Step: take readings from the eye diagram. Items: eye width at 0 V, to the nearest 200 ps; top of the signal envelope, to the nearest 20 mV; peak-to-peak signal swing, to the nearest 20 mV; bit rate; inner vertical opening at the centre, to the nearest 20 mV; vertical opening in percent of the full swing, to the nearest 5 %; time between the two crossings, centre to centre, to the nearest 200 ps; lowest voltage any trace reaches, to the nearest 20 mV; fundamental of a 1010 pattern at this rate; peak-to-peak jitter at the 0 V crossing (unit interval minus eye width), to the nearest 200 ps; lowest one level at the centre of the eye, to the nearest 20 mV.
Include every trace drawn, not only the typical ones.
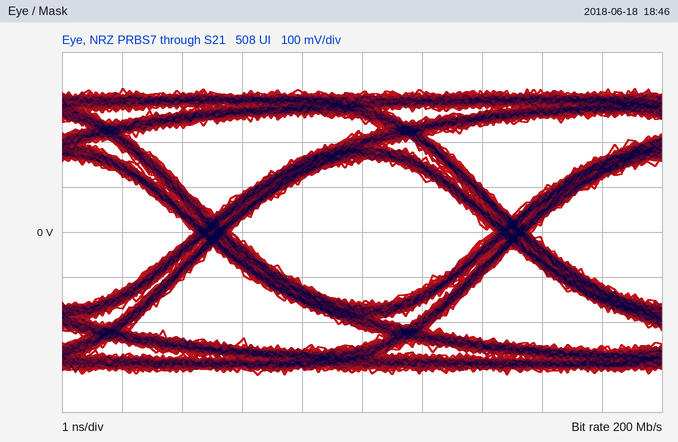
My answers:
4.4 ns
320 mV
640 mV
200 Mb/s
320 mV
50 %
5.0 ns
-320 mV
100 MHz
600 ps
160 mV
